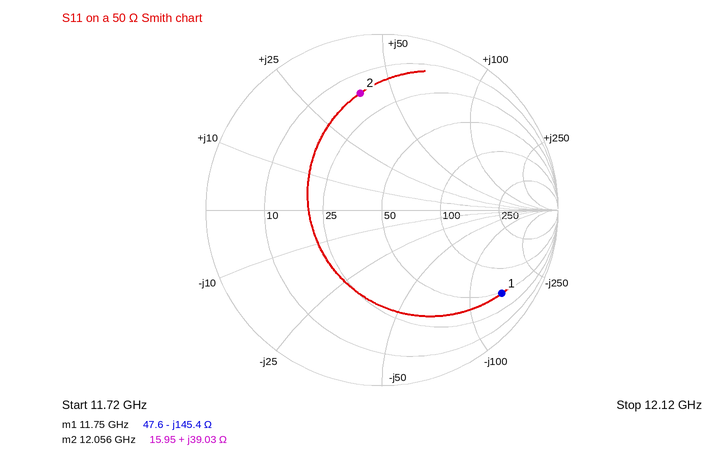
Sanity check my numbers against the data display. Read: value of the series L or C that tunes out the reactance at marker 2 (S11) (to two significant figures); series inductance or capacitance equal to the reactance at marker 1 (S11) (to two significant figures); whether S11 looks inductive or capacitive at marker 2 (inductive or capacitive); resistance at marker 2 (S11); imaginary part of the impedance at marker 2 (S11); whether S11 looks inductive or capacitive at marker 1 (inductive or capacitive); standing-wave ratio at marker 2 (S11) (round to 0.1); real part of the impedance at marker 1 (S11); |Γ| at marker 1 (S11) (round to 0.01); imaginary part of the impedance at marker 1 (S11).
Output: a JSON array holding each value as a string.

["340 fF", "93 fF", "inductive", "15.95 Ω", "+39.03 Ω", "capacitive", "5.2", "47.6 Ω", "0.83", "-145.4 Ω"]
